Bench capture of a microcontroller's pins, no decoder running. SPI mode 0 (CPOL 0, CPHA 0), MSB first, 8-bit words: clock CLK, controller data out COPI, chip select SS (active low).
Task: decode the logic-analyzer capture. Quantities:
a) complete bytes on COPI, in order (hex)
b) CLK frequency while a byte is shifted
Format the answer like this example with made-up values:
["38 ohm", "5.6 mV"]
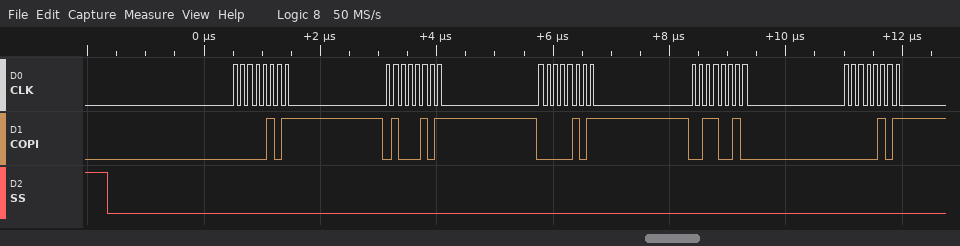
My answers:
["05 45 05 32 05", "8 MHz"]
